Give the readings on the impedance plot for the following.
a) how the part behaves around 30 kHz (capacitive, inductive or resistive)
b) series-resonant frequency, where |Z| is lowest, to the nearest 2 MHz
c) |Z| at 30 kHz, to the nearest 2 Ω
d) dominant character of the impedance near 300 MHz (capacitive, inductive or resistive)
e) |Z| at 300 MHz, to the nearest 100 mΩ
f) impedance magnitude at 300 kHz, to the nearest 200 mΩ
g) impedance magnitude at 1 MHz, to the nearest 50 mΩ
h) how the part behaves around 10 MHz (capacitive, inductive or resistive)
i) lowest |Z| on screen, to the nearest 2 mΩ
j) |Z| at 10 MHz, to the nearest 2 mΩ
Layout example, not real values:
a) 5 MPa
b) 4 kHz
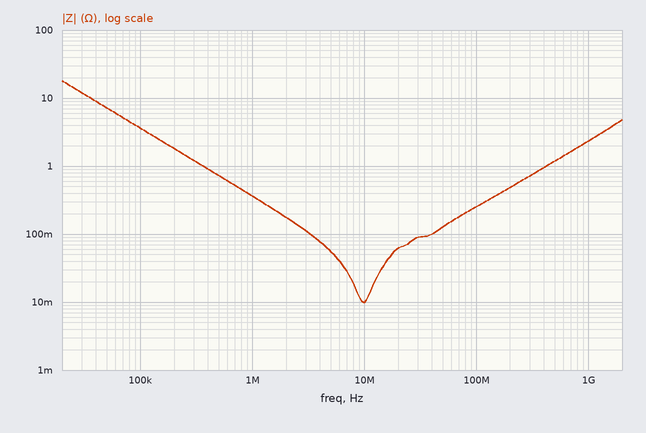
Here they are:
a) capacitive
b) 10 MHz
c) 12 Ω
d) inductive
e) 700 mΩ
f) 1.2 Ω
g) 350 mΩ
h) resistive
i) 10 mΩ
j) 10 mΩ
